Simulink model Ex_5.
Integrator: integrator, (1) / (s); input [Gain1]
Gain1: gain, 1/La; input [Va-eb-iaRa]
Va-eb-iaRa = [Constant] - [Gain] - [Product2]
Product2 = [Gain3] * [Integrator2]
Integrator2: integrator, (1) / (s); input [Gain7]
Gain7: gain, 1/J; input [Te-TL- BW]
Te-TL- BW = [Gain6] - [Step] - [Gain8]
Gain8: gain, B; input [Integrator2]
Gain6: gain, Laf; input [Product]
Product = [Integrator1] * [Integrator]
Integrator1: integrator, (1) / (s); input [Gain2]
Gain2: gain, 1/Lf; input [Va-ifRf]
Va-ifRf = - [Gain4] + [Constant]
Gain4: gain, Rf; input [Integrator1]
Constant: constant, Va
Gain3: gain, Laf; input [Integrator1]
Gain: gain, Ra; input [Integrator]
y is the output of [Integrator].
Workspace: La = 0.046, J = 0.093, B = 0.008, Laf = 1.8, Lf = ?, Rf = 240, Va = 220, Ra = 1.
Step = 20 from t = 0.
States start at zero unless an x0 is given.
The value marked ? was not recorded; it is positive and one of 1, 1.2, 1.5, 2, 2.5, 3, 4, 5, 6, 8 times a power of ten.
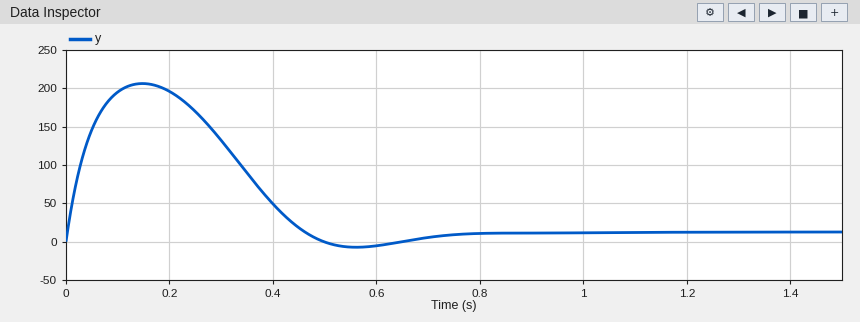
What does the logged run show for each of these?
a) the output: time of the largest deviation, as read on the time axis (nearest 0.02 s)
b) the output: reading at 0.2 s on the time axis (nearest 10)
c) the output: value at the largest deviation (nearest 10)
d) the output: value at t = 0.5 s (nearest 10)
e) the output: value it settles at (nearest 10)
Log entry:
0.14 s
200
210
0
10
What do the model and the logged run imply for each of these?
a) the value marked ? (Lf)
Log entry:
120
